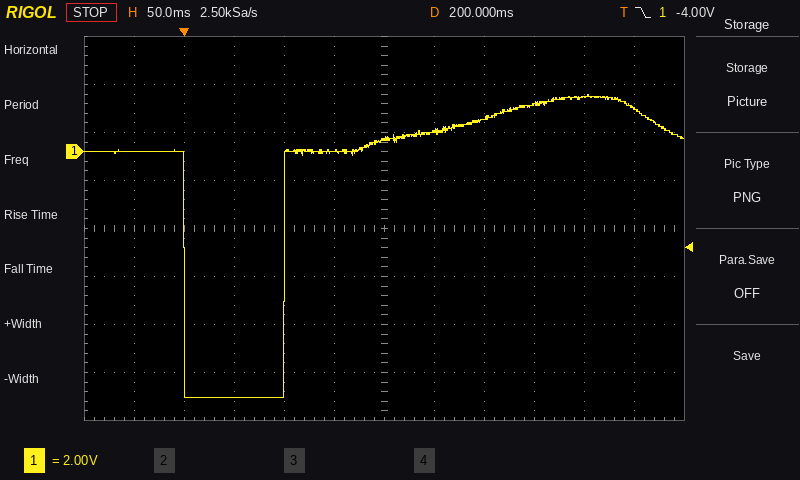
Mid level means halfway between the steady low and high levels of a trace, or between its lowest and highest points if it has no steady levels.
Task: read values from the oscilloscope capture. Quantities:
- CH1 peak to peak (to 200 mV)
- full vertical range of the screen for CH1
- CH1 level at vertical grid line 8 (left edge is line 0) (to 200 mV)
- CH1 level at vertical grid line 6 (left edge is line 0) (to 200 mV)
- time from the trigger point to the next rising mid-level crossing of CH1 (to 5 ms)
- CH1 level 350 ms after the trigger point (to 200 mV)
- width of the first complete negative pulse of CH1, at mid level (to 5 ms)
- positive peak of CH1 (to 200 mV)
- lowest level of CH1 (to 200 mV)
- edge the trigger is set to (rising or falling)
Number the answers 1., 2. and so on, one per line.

1. 12.6 V
2. 16 V
3. 1.4 V
4. 600 mV
5. 100 ms
6. 2.0 V
7. 100 ms
8. 2.4 V
9. -10.2 V
10. falling
